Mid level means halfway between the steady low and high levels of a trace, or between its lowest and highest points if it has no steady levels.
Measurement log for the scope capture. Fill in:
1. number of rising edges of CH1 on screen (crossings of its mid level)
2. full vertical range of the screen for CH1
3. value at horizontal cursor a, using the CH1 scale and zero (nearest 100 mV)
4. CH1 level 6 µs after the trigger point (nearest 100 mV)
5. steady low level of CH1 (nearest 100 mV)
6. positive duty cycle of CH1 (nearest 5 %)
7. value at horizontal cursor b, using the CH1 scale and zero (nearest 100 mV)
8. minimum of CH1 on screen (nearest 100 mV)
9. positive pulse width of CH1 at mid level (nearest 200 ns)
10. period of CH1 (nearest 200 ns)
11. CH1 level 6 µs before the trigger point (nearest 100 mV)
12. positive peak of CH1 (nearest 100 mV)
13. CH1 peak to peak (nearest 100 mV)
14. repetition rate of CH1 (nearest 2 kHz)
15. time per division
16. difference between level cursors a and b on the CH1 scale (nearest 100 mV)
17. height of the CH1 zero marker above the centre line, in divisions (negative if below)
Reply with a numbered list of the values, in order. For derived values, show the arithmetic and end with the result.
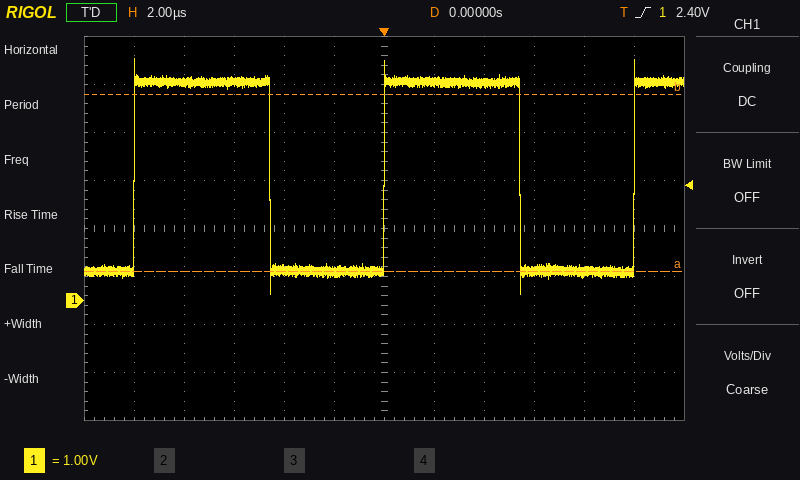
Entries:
1. 3
2. 8 V
3. 600 mV
4. 600 mV
5. 600 mV
6. 5.4 µs / 10.0 µs ≈ 54.0 %, so 55 % to the nearest 5 %
7. 4.3 V
8. 100 mV
9. 5.4 µs
10. 10.0 µs
11. 4.6 V
12. 5.0 V
13. 5.0 V − (100 mV) = 4.9 V
14. 1 / 10.0 µs ≈ 100 kHz
15. 2 µs
16. 3.7 V
17. -1.5 div
